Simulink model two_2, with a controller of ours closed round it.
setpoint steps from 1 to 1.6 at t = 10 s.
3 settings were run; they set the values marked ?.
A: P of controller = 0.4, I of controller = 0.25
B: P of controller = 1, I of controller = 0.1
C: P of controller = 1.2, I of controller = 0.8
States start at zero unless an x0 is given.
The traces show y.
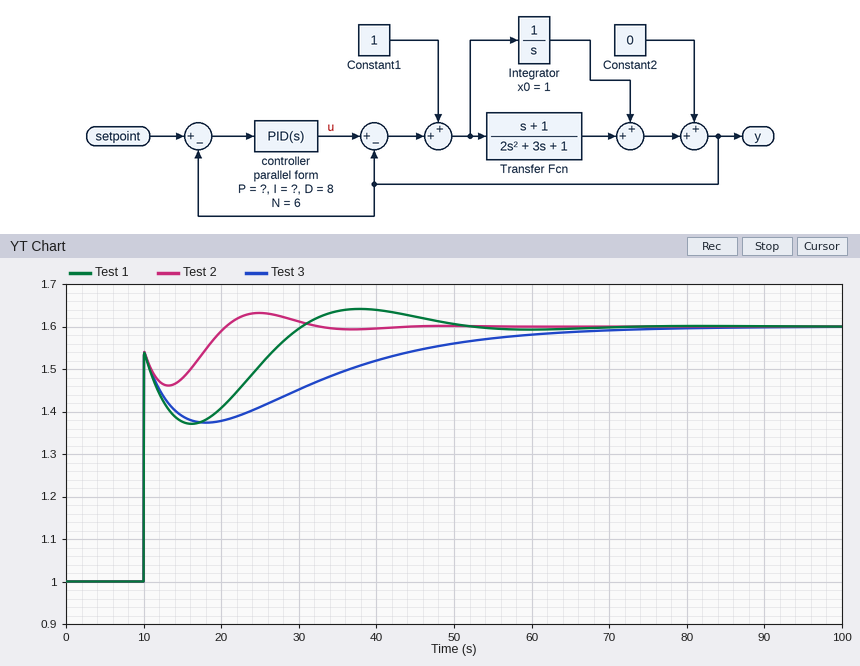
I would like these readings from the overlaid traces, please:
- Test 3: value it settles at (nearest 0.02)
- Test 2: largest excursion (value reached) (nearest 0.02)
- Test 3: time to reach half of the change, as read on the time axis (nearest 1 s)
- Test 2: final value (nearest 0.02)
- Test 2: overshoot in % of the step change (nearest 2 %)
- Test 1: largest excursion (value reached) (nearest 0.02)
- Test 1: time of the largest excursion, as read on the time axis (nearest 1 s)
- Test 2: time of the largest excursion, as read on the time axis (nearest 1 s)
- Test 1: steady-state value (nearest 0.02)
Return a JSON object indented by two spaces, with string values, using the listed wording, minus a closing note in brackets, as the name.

{
  "Test 3: value it settles at": "1.60",
  "Test 2: largest excursion (value reached)": "1.64",
  "Test 3: time to reach half of the change, as read on the time axis": "10 s",
  "Test 2: final value": "1.60",
  "Test 2: overshoot in % of the step change": "6 %",
  "Test 1: largest excursion (value reached)": "1.64",
  "Test 1: time of the largest excursion, as read on the time axis": "38 s",
  "Test 2: time of the largest excursion, as read on the time axis": "25 s",
  "Test 1: steady-state value": "1.60"
}
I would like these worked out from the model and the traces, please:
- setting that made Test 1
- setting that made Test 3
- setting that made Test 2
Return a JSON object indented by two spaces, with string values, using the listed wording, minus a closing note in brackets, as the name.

{
  "setting that made Test 1": "A",
  "setting that made Test 3": "B",
  "setting that made Test 2": "C"
}
